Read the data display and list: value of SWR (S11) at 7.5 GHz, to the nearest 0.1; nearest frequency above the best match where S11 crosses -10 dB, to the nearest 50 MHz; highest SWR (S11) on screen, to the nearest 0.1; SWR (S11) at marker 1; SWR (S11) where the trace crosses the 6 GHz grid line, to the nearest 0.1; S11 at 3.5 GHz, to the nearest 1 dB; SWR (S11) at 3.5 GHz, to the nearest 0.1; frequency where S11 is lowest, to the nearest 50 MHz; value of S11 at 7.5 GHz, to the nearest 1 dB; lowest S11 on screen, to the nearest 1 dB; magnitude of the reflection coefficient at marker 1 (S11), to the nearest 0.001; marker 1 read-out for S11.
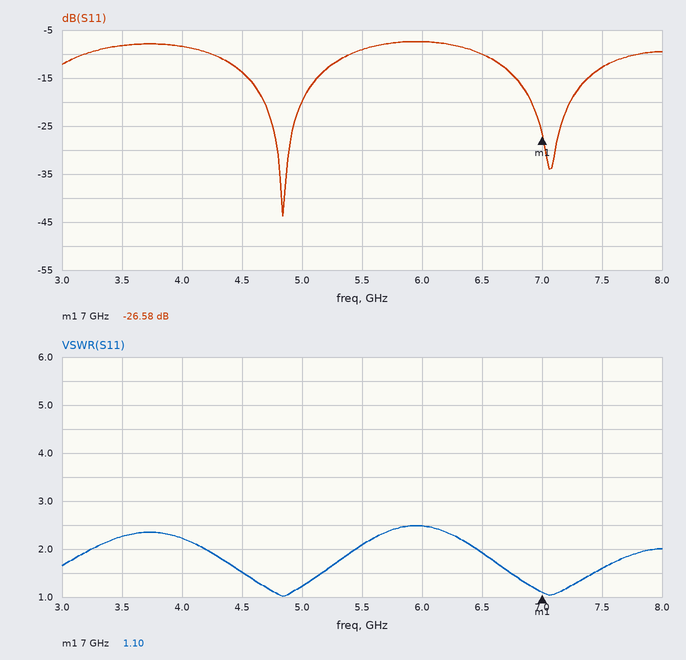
1.6
5.40 GHz
2.5
1.10
2.5
-8 dB
2.3
4.85 GHz
-13 dB
-44 dB
0.047
-26.58 dB
